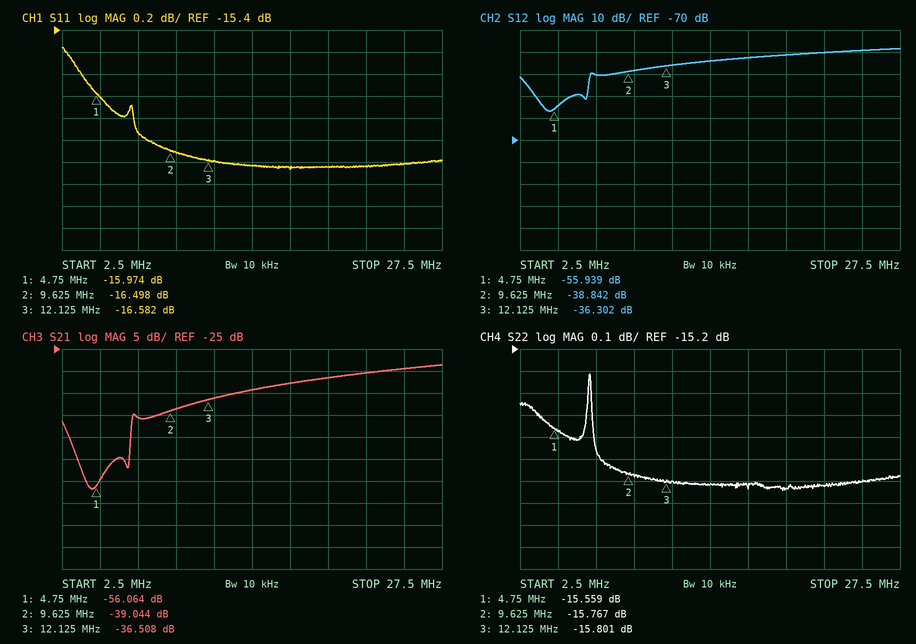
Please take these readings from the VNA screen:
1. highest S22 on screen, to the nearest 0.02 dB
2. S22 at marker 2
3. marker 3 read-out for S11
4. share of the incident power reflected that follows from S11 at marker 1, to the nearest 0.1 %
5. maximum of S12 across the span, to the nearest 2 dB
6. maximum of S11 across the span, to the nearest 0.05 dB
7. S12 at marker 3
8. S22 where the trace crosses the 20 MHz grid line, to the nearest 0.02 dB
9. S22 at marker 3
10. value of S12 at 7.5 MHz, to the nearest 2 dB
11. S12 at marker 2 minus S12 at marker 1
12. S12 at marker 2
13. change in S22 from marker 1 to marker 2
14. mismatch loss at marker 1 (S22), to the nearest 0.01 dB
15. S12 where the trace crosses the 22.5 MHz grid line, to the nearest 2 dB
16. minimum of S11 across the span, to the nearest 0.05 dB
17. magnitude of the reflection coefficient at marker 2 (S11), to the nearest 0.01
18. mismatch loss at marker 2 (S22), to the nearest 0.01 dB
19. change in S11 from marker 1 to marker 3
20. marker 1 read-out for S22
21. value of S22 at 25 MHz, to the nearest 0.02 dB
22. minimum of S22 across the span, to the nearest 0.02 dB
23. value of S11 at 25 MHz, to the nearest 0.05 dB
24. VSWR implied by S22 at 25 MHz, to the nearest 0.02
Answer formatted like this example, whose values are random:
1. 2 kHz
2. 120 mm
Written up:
1. -15.32 dB
2. -15.767 dB
3. -16.582 dB
4. 2.5 %
5. -28 dB
6. -15.55 dB
7. -36.302 dB
8. -15.84 dB
9. -15.801 dB
10. -40 dB
11. 17.097 dB
12. -38.842 dB
13. -0.208 dB
14. 0.12 dB
15. -30 dB
16. -16.65 dB
17. 0.15
18. 0.12 dB
19. -0.608 dB
20. -15.559 dB
21. -15.80 dB
22. -15.84 dB
23. -16.60 dB
24. 1.38
